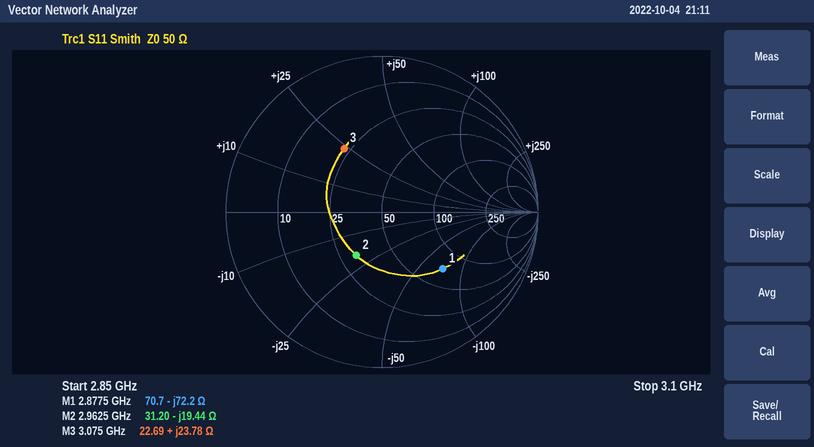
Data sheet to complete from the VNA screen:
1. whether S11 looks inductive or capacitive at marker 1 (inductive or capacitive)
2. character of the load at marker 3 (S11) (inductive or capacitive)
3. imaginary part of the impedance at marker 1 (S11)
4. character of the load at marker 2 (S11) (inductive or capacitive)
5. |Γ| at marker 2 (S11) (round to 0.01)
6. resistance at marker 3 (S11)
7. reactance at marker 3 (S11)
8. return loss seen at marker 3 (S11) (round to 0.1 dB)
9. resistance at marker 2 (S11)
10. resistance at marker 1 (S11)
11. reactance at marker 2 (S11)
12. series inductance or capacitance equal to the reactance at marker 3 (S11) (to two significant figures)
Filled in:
capacitive
inductive
-72.2 Ω
capacitive
0.32
22.69 Ω
+23.78 Ω
6.5 dB
31.20 Ω
70.7 Ω
-19.44 Ω
1.2 nH
